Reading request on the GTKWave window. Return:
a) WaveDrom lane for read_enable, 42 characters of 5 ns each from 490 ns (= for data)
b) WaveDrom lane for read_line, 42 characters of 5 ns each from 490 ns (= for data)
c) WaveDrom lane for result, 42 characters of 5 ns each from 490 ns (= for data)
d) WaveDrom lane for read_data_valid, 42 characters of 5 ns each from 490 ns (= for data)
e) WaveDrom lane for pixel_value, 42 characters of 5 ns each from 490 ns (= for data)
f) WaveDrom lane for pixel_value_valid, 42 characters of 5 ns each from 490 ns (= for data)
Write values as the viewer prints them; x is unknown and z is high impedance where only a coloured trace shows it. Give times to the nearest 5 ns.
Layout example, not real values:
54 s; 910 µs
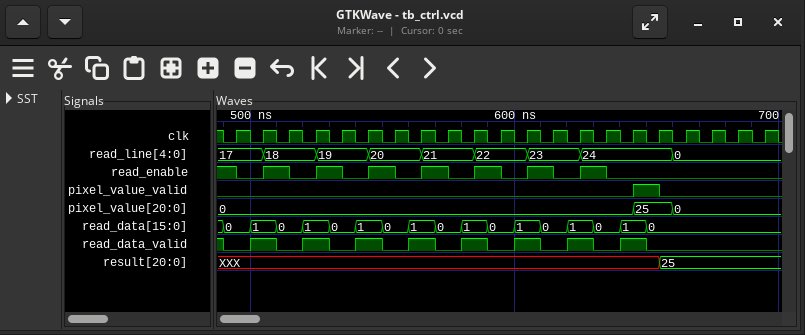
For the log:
{name: 'read_enable', wave: '10.1.0.1.0.1.0.1.0.1.0.1.0.1.0............'}; {name: 'read_line', wave: '=..=...=...=...=...=...=...=......=.......', data: '17 18 19 20 21 22 23 24 0'}; {name: 'result', wave: 'x................................=........', data: '25'}; {name: 'read_data_valid', wave: '0.1.0.1.0.1.0.1.0.1.0.1.0.1.0.1.0.........'}; {name: 'pixel_value', wave: '=..............................=..=.......', data: '0 25 0'}; {name: 'pixel_value_valid', wave: '0..............................1.0........'}
